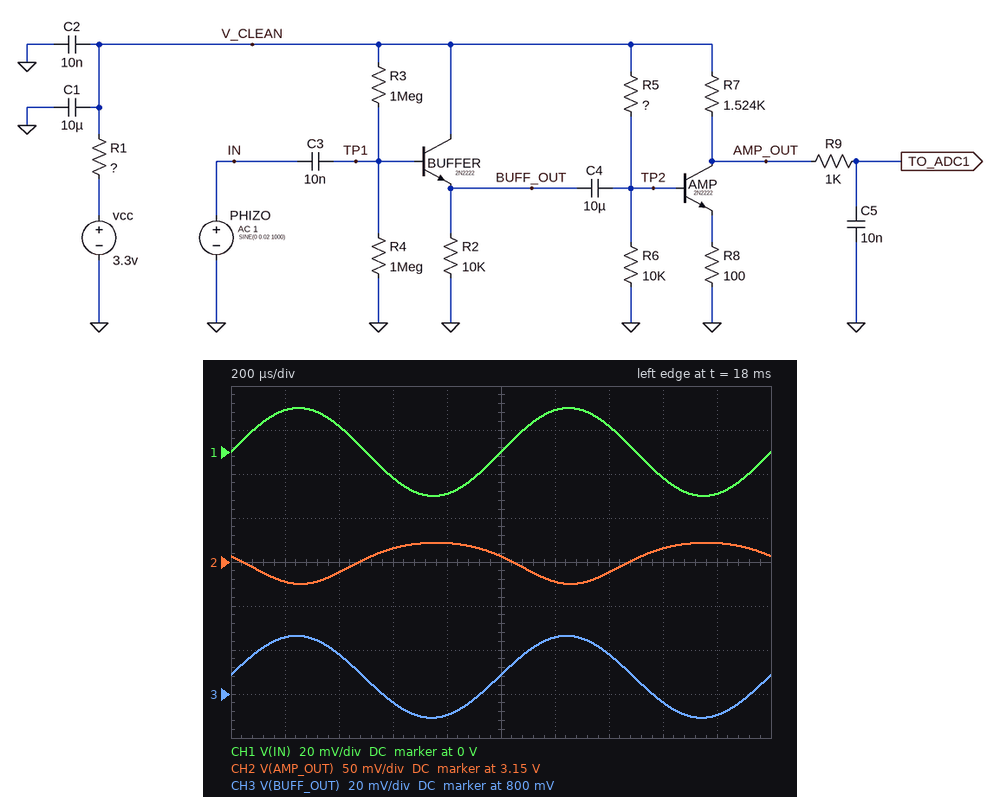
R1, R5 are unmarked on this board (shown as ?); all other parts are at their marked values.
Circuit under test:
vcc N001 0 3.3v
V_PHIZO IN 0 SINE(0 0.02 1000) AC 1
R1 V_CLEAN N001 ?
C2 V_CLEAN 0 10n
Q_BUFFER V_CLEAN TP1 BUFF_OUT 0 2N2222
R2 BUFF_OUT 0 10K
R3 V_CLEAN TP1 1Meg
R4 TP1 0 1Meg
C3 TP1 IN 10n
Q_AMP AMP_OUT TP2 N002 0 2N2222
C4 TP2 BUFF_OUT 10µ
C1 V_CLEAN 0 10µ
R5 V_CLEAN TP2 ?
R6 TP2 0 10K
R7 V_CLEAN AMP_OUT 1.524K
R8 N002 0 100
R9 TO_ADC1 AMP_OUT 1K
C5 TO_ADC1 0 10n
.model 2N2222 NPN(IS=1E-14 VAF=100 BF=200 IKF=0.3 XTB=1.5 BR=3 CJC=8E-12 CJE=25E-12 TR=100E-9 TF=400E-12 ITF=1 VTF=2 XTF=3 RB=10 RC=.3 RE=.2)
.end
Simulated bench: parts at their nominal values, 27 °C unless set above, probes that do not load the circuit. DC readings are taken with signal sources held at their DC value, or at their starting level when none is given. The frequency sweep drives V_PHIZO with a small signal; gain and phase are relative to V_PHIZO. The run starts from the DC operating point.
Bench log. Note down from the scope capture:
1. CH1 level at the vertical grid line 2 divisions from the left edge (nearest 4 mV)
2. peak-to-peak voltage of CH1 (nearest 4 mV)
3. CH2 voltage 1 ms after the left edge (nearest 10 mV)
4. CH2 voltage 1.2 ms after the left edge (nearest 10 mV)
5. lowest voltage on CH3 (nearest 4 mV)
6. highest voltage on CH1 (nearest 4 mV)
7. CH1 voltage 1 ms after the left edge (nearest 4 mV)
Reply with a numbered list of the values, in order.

1. 12 mV
2. 40 mV
3. 3.16 V
4. 3.13 V
5. 788 mV
6. 20 mV
7. 0 V
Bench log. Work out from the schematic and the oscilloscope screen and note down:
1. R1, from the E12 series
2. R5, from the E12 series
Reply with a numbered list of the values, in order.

1. 680 Ω
2. 47 kΩ
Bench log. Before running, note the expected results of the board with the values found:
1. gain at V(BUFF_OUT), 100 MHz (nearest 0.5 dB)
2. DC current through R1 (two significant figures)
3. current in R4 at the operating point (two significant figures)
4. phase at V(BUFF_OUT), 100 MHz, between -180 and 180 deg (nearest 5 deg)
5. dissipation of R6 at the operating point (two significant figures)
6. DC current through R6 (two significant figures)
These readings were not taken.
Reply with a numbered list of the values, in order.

1. -2.5 dB
2. 160 µA
3. 1.4 µA
4. 10 deg
5. 31 µW
6. 56 µA
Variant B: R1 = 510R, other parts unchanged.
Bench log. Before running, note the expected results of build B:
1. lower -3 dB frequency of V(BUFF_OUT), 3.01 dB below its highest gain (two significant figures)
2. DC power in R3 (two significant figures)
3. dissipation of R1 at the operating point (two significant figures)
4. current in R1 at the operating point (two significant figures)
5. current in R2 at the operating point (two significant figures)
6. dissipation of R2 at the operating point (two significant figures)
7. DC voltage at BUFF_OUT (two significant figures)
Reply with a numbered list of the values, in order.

1. 48 Hz
2. 3.3 µW
3. 14 µW
4. 170 µA
5. 82 µA
6. 67 µW
7. 820 mV
